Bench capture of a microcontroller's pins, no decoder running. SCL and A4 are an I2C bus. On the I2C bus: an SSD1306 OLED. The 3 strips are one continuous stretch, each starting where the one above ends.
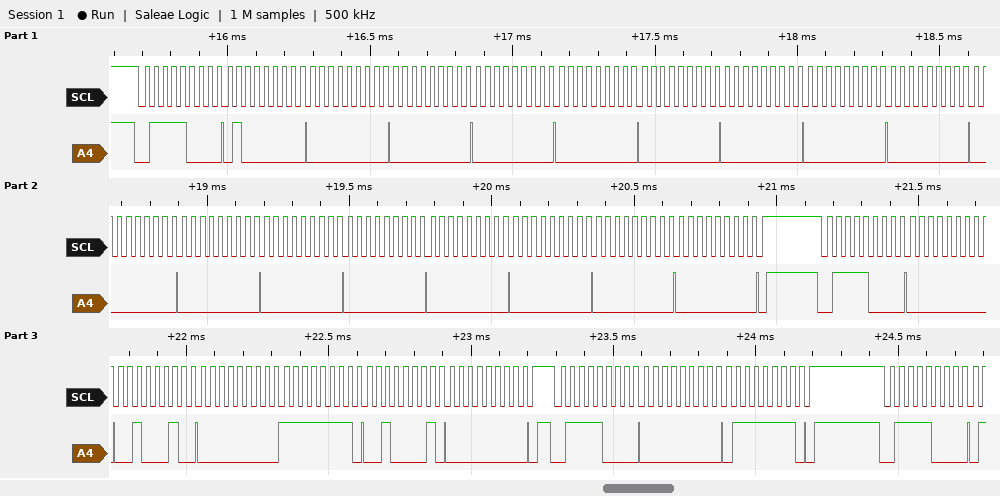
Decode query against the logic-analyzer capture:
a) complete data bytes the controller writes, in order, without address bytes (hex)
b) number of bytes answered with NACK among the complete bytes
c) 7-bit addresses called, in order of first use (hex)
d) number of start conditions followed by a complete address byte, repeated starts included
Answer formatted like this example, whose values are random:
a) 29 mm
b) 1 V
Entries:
a) 40 00 00 00 00 00 00 00 00 00 00 00 00 00 00 00 00 00 22 00 FF 21 00 00 7F
b) 0
c) 0x3C
d) 4
